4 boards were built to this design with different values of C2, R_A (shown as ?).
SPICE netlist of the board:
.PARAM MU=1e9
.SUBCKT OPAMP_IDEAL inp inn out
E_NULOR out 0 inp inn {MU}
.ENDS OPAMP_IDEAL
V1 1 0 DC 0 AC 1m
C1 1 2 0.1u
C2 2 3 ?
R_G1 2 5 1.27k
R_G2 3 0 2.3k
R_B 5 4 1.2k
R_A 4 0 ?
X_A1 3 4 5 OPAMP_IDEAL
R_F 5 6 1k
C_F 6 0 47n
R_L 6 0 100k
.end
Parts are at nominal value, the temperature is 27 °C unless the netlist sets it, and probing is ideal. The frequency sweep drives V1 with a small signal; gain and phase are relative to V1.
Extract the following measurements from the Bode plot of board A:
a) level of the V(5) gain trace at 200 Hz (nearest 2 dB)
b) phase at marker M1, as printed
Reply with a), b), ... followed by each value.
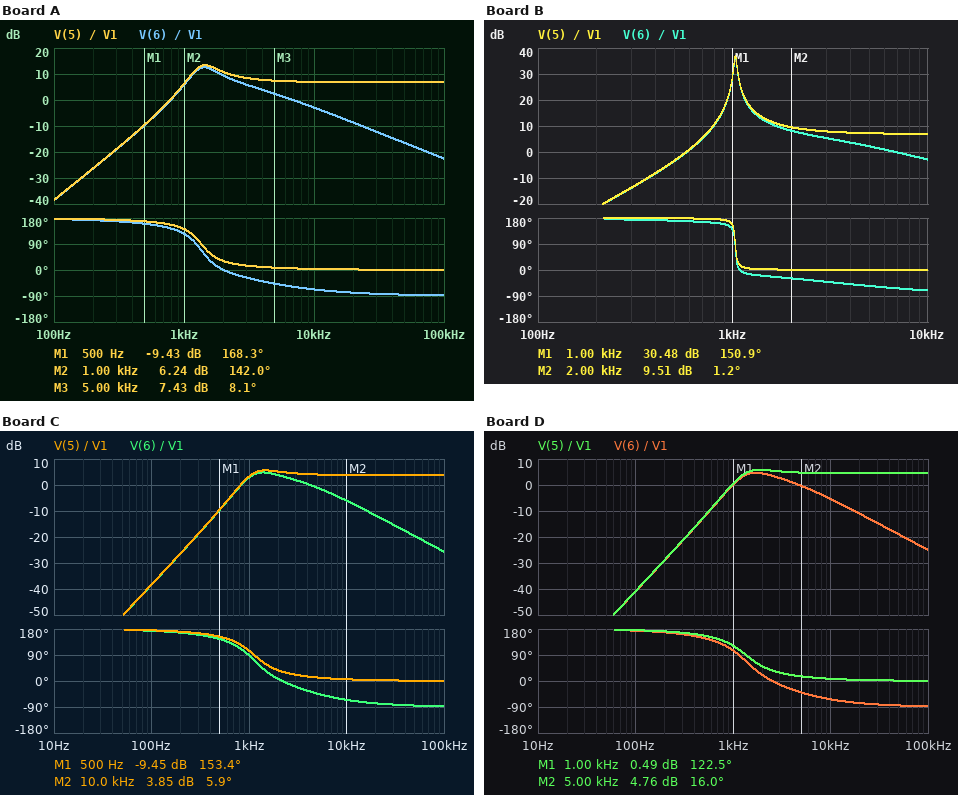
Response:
a) -26 dB
b) 168.3 deg
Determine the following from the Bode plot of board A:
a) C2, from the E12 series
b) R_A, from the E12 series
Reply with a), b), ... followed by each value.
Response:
a) 47 nF
b) 1 kΩ
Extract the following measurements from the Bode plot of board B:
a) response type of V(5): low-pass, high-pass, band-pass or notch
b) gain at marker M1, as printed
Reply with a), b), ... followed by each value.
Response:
a) high-pass
b) 30.48 dB
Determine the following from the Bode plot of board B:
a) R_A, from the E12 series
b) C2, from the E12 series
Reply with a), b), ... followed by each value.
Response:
a) 1 kΩ
b) 82 nF
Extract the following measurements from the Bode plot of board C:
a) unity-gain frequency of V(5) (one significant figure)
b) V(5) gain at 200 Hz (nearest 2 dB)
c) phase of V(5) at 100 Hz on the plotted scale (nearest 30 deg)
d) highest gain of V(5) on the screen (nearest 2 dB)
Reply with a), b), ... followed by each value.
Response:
a) 800 Hz
b) -26 dB
c) 180 deg
d) 6 dB
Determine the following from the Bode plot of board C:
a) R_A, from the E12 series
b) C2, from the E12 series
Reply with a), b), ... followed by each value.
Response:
a) 2.2 kΩ
b) 68 nF
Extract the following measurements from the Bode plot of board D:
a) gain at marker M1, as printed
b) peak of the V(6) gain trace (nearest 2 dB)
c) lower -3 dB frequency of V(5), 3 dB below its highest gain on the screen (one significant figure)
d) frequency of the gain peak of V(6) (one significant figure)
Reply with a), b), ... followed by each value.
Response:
a) 0.49 dB
b) 4 dB
c) 1 kHz
d) 2 kHz
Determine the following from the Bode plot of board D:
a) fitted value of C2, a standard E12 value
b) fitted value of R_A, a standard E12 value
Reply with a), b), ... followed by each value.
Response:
a) 47 nF
b) 1.8 kΩ
